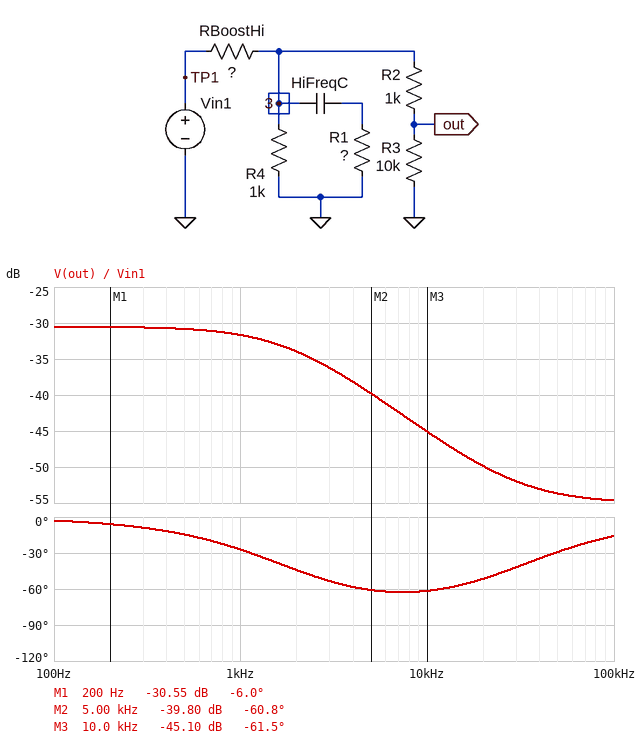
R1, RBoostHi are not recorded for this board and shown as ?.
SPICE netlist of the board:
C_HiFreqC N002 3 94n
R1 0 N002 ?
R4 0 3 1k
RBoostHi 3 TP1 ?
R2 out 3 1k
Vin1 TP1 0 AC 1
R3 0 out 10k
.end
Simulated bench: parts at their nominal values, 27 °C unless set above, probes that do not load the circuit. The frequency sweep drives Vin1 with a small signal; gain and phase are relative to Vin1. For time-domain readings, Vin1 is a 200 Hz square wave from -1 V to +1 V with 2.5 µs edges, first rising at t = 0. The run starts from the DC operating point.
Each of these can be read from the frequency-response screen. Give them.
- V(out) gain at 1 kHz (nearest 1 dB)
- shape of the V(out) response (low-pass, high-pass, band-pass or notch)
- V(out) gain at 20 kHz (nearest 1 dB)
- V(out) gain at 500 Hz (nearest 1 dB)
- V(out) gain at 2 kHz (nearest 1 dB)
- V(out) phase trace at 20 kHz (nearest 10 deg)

-32 dB
low-pass
-50 dB
-31 dB
-34 dB
-50 deg
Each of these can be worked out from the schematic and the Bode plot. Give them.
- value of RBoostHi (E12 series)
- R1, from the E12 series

27 kΩ
56 Ω
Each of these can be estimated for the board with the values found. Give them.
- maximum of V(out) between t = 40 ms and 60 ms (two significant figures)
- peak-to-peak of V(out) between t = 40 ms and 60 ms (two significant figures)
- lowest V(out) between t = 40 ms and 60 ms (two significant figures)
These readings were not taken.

30 mV
60 mV
-30 mV
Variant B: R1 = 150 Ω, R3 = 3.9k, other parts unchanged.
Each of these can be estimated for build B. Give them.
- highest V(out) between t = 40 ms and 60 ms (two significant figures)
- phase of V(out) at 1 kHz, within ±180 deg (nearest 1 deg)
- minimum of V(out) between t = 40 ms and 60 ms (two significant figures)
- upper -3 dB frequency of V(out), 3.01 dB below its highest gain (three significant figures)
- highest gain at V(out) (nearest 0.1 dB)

24 mV
-24 deg
-24 mV
1.82 kHz
-32.5 dB
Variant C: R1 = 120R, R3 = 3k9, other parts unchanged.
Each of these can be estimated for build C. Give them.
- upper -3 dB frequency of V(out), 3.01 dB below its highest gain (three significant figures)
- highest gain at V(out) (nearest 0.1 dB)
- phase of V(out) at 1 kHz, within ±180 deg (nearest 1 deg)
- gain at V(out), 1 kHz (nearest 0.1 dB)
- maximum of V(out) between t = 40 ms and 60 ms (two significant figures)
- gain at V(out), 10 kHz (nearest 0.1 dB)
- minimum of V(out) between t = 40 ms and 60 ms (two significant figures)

1.86 kHz
-32.5 dB
-25 deg
-33.6 dB
24 mV
-45.6 dB
-24 mV
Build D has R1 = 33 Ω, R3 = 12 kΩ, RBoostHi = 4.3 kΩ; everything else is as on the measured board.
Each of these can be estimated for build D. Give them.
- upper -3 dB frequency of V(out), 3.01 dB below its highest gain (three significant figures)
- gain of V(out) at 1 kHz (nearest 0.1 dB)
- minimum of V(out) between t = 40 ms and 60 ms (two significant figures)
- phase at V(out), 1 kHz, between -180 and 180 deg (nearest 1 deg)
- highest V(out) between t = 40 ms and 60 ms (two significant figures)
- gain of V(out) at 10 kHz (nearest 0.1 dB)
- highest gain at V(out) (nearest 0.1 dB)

2.13 kHz
-16.6 dB
-160 mV
-24 deg
160 mV
-29.2 dB
-15.7 dB
